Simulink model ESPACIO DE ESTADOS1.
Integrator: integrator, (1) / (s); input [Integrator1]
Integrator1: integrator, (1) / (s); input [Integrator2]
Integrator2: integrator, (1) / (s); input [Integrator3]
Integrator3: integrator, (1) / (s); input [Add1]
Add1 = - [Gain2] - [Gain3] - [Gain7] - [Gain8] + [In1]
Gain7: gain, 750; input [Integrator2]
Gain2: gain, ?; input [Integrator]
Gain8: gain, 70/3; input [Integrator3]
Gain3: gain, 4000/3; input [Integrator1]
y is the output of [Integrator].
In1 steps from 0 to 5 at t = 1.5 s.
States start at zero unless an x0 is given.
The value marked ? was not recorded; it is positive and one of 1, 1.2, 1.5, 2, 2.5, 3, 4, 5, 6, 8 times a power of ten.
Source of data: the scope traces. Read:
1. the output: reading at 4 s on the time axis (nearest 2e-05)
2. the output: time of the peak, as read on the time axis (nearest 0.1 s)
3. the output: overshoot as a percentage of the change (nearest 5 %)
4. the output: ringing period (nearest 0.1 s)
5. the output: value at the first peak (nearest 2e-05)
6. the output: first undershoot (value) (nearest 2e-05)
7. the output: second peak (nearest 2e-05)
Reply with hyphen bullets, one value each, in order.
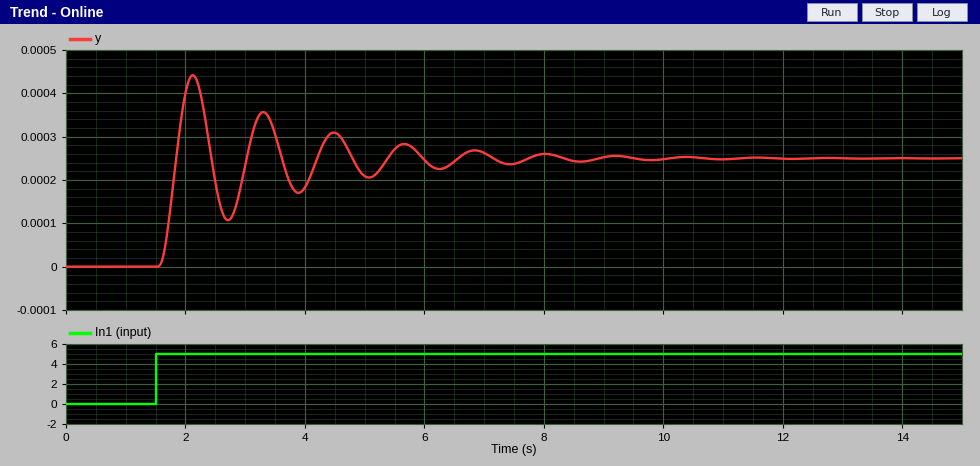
- 0.00018
- 2.1 s
- 75 %
- 1.2 s
- 0.00044
- 0.00010
- 0.00036
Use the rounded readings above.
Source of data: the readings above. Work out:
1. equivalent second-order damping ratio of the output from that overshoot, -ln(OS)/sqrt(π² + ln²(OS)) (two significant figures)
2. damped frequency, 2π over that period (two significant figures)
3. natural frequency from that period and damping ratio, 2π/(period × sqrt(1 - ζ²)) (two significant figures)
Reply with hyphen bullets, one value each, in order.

- 0.091
- 5.2 rad/s
- 5.3 rad/s
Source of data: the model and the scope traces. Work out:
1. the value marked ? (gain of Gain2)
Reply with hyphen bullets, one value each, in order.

- 20000
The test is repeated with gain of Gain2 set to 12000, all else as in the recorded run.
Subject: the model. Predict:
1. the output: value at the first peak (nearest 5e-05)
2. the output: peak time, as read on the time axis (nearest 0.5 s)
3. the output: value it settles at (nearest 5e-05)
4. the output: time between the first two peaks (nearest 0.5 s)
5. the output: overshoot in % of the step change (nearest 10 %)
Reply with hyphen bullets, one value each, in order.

- 0.00065
- 2.5 s
- 0.00040
- 1.5 s
- 60 %
